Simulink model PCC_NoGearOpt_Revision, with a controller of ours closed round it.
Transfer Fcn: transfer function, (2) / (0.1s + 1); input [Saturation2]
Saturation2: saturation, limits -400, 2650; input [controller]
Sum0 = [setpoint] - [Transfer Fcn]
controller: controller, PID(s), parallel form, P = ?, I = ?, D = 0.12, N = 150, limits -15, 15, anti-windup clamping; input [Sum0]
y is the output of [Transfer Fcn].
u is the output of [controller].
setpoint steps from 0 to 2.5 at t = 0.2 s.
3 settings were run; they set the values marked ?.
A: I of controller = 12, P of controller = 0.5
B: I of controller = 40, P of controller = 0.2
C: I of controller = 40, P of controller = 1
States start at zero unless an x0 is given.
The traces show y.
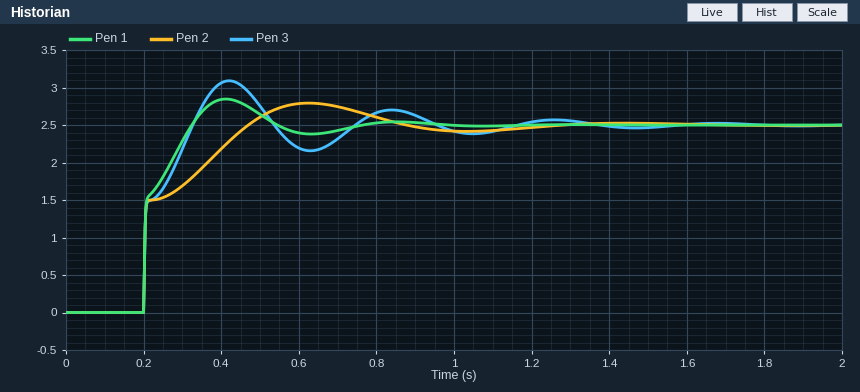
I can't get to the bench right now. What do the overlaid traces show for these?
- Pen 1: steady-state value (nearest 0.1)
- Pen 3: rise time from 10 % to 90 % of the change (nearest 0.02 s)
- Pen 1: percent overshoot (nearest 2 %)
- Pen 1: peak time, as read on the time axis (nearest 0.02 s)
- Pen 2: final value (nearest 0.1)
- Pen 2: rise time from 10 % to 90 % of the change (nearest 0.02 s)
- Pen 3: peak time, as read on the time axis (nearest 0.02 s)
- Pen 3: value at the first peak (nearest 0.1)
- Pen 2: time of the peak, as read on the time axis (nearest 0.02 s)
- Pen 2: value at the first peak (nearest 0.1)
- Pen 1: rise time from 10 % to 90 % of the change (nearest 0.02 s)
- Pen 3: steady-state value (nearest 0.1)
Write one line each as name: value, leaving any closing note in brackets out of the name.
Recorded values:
Pen 1: steady-state value: 2.5
Pen 3: rise time from 10 % to 90 % of the change: 0.10 s
Pen 1: percent overshoot: 14 %
Pen 1: peak time, as read on the time axis: 0.42 s
Pen 2: final value: 2.5
Pen 2: rise time from 10 % to 90 % of the change: 0.22 s
Pen 3: peak time, as read on the time axis: 0.42 s
Pen 3: value at the first peak: 3.1
Pen 2: time of the peak, as read on the time axis: 0.62 s
Pen 2: value at the first peak: 2.8
Pen 1: rise time from 10 % to 90 % of the change: 0.10 s
Pen 3: steady-state value: 2.5
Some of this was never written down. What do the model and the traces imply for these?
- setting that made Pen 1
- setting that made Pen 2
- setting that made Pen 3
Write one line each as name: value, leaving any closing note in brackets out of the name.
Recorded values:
setting that made Pen 1: C
setting that made Pen 2: A
setting that made Pen 3: B
